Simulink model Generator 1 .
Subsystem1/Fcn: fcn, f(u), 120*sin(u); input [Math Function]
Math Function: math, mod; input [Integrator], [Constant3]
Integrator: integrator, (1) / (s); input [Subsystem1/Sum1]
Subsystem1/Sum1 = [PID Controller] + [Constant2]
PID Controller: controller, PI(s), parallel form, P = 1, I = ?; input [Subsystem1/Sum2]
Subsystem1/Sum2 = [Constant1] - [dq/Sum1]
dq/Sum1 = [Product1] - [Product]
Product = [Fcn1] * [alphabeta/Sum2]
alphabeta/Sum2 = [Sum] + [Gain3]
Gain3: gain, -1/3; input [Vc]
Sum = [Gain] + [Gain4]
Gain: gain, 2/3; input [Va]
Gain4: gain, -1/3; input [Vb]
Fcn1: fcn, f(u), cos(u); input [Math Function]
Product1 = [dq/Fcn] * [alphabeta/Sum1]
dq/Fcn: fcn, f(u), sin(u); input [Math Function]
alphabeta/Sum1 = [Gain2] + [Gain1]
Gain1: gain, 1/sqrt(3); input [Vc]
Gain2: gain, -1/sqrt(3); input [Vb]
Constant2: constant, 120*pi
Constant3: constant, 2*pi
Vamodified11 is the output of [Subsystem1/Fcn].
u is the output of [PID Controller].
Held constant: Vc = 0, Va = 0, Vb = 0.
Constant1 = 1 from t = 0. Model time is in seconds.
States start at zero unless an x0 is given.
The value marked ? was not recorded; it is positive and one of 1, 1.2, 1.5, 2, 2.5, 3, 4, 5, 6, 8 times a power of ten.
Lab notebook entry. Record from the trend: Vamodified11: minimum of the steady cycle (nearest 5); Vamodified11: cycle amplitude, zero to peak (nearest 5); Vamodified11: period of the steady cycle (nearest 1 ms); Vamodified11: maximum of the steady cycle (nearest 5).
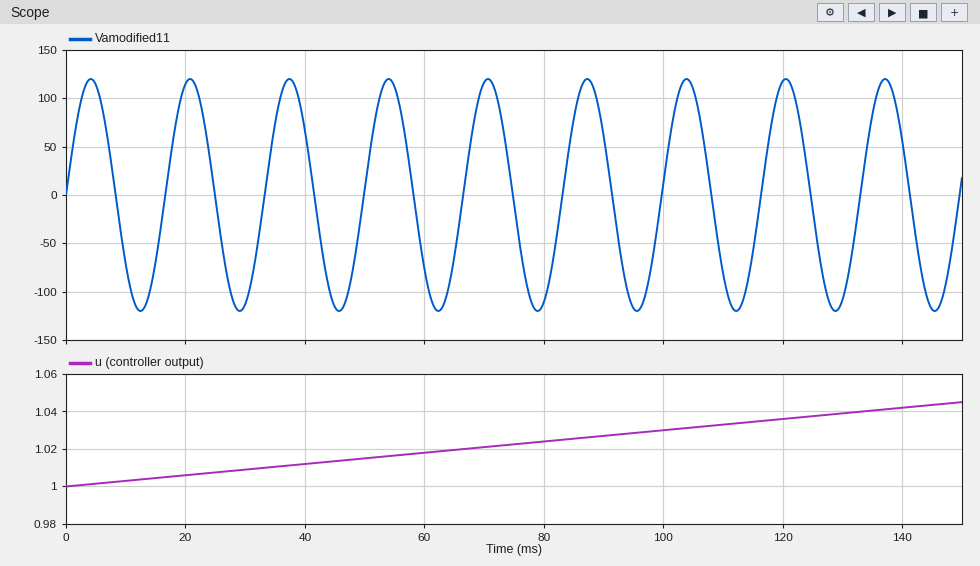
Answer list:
-120
120
17 ms
120
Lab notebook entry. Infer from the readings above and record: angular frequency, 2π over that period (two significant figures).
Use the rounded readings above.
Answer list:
0.37 rad/ms
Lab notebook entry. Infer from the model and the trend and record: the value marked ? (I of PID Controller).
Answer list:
0.3
